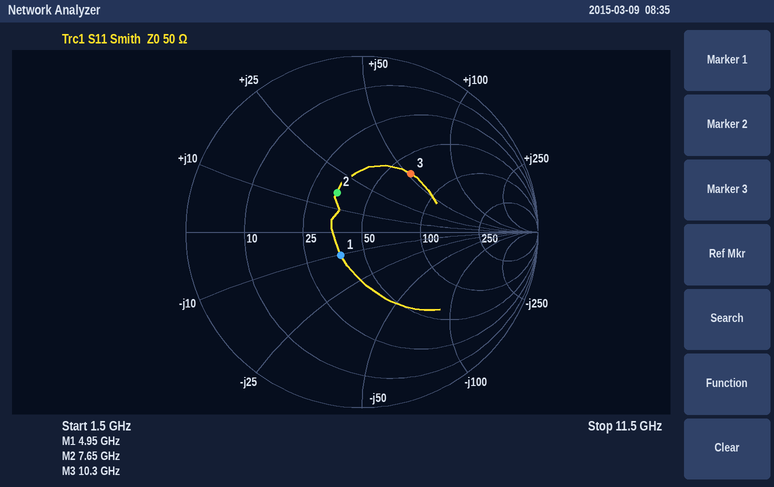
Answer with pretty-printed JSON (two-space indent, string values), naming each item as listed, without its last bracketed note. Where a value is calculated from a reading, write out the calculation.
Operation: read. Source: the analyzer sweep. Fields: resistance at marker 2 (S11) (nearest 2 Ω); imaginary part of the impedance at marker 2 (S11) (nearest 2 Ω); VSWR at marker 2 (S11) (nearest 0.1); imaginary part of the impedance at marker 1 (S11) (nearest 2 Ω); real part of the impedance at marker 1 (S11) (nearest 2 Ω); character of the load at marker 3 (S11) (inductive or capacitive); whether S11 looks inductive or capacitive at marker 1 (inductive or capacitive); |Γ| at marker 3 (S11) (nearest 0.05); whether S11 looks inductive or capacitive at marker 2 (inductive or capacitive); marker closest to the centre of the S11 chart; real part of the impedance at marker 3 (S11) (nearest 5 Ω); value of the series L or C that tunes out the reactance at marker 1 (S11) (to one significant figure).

{
  "resistance at marker 2 (S11)": "34 Ω",
  "imaginary part of the impedance at marker 2 (S11)": "+16 Ω",
  "VSWR at marker 2 (S11)": "1.7",
  "imaginary part of the impedance at marker 1 (S11)": "-10 Ω",
  "real part of the impedance at marker 1 (S11)": "38 Ω",
  "character of the load at marker 3 (S11)": "inductive",
  "whether S11 looks inductive or capacitive at marker 1": "capacitive",
  "|Γ| at marker 3 (S11)": "0.45",
  "whether S11 looks inductive or capacitive at marker 2": "inductive",
  "marker closest to the centre of the S11 chart": "marker 1",
  "real part of the impedance at marker 3 (S11)": "65 Ω",
  "value of the series L or C that tunes out the reactance at marker 1 (S11)": "L = 10 Ω/(2π × 4.95 GHz) ≈ 322 pH, so 300 pH to one significant figure"
}
